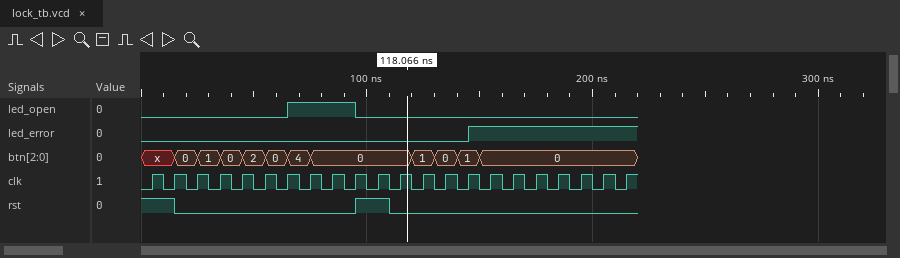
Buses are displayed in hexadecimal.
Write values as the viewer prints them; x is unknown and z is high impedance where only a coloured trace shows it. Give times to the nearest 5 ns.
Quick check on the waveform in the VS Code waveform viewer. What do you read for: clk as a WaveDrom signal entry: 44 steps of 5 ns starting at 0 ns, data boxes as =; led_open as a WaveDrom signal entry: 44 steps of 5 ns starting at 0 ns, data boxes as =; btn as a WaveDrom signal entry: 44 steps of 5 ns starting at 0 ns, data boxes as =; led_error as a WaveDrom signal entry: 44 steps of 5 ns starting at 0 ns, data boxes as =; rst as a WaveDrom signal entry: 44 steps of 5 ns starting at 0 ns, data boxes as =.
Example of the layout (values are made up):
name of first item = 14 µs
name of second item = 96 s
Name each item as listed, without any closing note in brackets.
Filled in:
clk as a WaveDrom signal entry: 44 steps of 5 ns starting at 0 ns, data boxes as = = {name: 'clk', wave: '01010101010101010101010101010101010101010101'}
led_open as a WaveDrom signal entry: 44 steps of 5 ns starting at 0 ns, data boxes as = = {name: 'led_open', wave: '0............1.....0........................'}
btn as a WaveDrom signal entry: 44 steps of 5 ns starting at 0 ns, data boxes as = = {name: 'btn', wave: 'x..=.=.=.=.=.=.=........=.=.=.=.............', data: '0 1 0 2 0 4 0 1 0 1 0'}
led_error as a WaveDrom signal entry: 44 steps of 5 ns starting at 0 ns, data boxes as = = {name: 'led_error', wave: '0............................1..............'}
rst as a WaveDrom signal entry: 44 steps of 5 ns starting at 0 ns, data boxes as = = {name: 'rst', wave: '1..0...............1..0.....................'}
